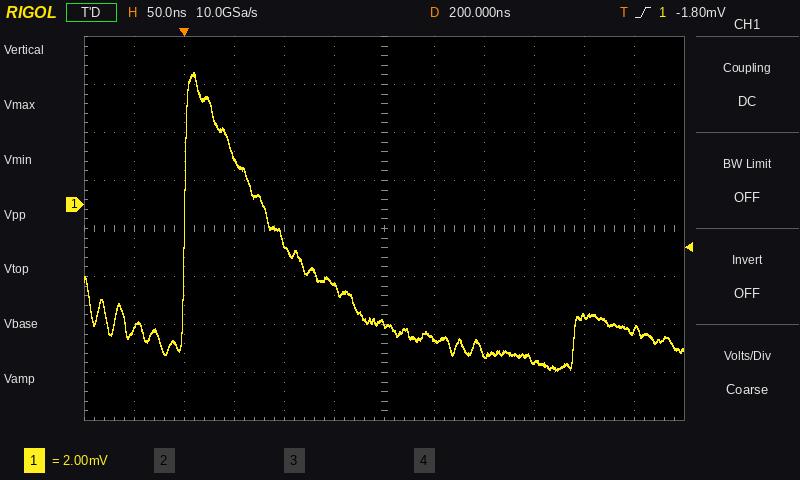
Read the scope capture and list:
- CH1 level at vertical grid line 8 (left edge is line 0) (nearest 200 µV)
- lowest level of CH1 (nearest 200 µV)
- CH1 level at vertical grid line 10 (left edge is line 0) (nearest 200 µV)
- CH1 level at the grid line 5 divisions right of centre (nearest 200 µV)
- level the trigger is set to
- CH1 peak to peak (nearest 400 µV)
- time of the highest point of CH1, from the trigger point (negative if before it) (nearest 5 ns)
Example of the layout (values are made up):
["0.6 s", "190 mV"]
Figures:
["-6.2 mV", "-7.0 mV", "-4.6 mV", "-5.2 mV", "-1.80 mV", "12.4 mV", "+10 ns"]
